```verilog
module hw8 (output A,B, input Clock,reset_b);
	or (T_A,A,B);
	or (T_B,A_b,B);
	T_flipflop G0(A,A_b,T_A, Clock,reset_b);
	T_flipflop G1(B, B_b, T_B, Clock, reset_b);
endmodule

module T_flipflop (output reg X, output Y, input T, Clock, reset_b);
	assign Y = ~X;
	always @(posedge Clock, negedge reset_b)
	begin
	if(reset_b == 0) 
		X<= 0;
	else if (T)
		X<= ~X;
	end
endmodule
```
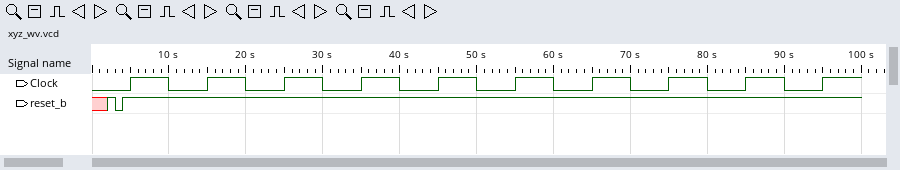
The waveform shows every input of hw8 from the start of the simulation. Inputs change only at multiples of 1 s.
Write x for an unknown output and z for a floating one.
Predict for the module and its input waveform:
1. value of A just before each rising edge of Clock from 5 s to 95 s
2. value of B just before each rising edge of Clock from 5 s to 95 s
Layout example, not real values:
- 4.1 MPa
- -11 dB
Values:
- 0 0 1 0 0 1 0 0 1 0
- 0 1 0 0 1 0 0 1 0 0
